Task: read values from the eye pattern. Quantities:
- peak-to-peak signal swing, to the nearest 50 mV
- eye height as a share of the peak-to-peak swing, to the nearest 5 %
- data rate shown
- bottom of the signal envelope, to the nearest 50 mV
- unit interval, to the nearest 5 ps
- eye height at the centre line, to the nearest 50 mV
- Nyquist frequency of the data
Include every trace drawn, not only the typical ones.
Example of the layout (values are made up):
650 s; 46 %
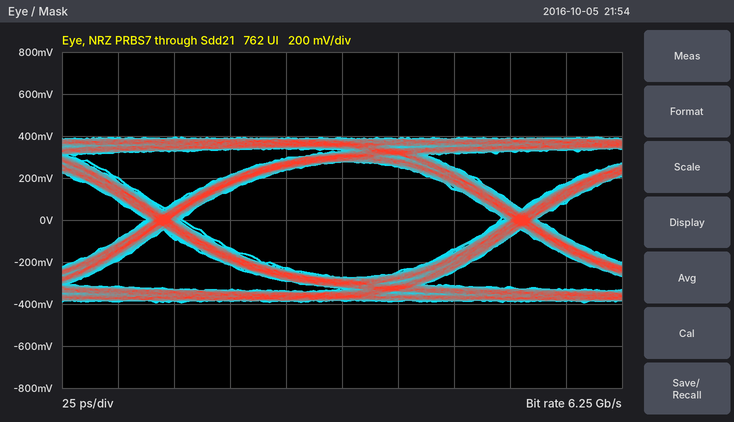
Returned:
800 mV; 70 %; 6.25 Gb/s; -400 mV; 160 ps; 550 mV; 3.125 GHz
